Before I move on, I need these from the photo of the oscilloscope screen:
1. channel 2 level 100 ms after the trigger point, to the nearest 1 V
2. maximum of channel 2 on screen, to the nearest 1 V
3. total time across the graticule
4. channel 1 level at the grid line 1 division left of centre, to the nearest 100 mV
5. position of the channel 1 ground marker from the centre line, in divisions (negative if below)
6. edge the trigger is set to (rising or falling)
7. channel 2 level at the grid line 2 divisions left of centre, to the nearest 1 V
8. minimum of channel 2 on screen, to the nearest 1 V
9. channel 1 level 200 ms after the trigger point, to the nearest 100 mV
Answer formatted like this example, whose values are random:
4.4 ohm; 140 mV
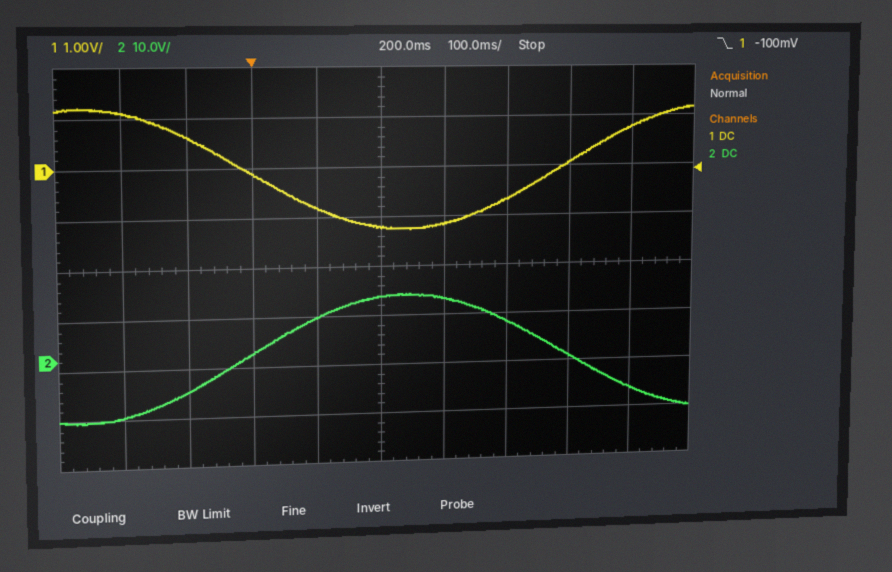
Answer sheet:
8 V; 12 V; 1 s; -800 mV; +2.0 div; falling; 1 V; -12 V; -1.2 V
